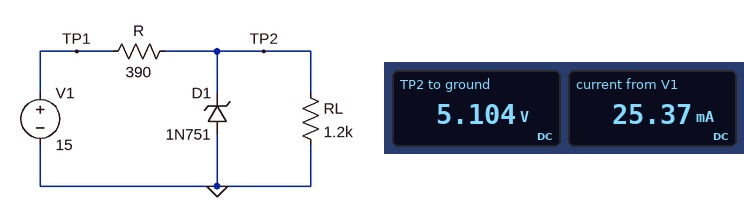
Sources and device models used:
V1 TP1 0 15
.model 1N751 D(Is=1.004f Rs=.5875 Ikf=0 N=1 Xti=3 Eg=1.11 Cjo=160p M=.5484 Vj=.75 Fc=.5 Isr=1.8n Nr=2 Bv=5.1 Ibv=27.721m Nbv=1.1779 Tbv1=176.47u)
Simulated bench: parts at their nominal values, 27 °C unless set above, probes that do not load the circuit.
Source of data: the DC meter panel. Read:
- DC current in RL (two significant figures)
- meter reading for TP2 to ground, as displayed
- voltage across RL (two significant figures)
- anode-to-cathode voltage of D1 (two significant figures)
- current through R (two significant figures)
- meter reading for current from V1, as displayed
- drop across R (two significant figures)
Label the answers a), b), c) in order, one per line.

a) 4.3 mA
b) 5.104 V
c) 5.1 V
d) -5.1 V
e) 25 mA
f) 25.37 mA
g) 9.9 V
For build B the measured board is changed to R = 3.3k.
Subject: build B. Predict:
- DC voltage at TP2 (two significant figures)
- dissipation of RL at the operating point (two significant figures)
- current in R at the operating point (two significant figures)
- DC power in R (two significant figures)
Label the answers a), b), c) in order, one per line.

a) 4.0 V
b) 13 mW
c) 3.3 mA
d) 37 mW
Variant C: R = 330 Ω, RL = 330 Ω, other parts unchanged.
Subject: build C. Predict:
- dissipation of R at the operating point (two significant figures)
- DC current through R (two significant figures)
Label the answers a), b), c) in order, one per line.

a) 300 mW
b) 30 mA
